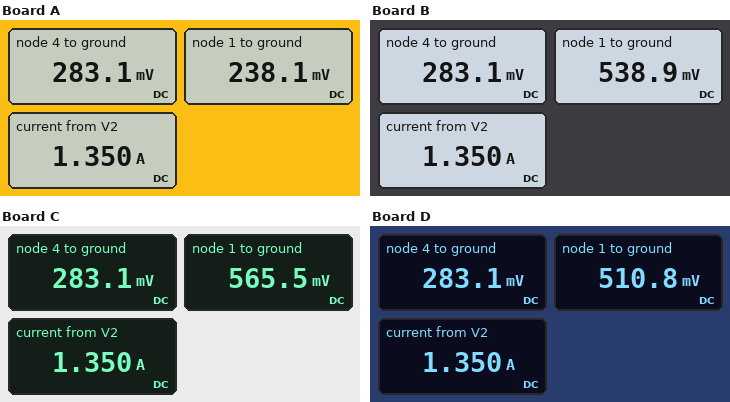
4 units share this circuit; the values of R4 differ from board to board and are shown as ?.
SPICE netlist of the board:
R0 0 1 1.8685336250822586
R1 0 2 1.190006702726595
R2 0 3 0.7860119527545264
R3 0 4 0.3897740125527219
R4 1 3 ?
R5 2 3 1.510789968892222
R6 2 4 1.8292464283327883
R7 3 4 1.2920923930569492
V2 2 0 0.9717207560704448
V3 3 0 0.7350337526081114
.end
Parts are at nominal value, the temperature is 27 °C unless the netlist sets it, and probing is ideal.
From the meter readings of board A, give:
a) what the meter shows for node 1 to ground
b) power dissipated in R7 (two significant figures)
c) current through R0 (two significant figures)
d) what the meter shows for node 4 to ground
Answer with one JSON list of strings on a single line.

["238.1 mV", "160 mW", "130 mA", "283.1 mV"]
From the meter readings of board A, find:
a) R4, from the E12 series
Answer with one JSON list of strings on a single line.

["3.9 Ω"]
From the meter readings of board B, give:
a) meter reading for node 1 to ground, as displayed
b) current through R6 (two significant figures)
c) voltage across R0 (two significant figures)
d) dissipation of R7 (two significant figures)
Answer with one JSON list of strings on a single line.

["538.9 mV", "380 mA", "540 mV", "160 mW"]
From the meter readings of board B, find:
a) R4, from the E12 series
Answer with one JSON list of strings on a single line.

["0.68 Ω"]
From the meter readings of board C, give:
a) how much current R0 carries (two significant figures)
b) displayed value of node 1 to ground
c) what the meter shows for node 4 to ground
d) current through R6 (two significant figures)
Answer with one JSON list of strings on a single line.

["300 mA", "565.5 mV", "283.1 mV", "380 mA"]
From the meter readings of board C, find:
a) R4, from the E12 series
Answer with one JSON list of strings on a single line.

["0.56 Ω"]
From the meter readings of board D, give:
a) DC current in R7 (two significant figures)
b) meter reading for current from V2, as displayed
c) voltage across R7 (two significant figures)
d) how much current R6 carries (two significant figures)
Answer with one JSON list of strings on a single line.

["350 mA", "1.350 A", "450 mV", "380 mA"]
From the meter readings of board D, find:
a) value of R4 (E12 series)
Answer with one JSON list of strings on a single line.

["0.82 Ω"]
